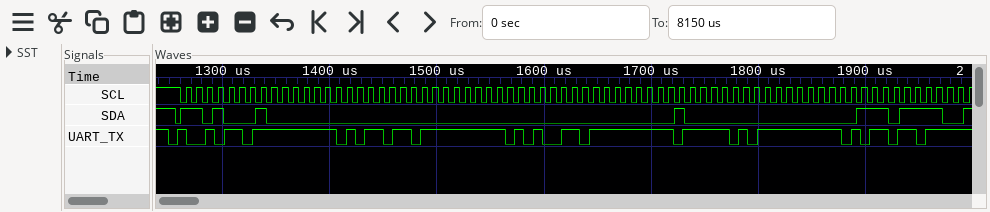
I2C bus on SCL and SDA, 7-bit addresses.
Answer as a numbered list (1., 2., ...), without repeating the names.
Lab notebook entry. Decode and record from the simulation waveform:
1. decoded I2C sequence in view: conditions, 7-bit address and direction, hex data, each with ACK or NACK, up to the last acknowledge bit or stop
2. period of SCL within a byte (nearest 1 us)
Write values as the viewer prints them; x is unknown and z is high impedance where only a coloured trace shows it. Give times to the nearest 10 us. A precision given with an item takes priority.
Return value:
1. start, address 68 read ACK, 00 ACK, 00 ACK, 00 ACK, 00 ACK, 40 ACK, 00 ACK, EF ACK
2. 10 us
